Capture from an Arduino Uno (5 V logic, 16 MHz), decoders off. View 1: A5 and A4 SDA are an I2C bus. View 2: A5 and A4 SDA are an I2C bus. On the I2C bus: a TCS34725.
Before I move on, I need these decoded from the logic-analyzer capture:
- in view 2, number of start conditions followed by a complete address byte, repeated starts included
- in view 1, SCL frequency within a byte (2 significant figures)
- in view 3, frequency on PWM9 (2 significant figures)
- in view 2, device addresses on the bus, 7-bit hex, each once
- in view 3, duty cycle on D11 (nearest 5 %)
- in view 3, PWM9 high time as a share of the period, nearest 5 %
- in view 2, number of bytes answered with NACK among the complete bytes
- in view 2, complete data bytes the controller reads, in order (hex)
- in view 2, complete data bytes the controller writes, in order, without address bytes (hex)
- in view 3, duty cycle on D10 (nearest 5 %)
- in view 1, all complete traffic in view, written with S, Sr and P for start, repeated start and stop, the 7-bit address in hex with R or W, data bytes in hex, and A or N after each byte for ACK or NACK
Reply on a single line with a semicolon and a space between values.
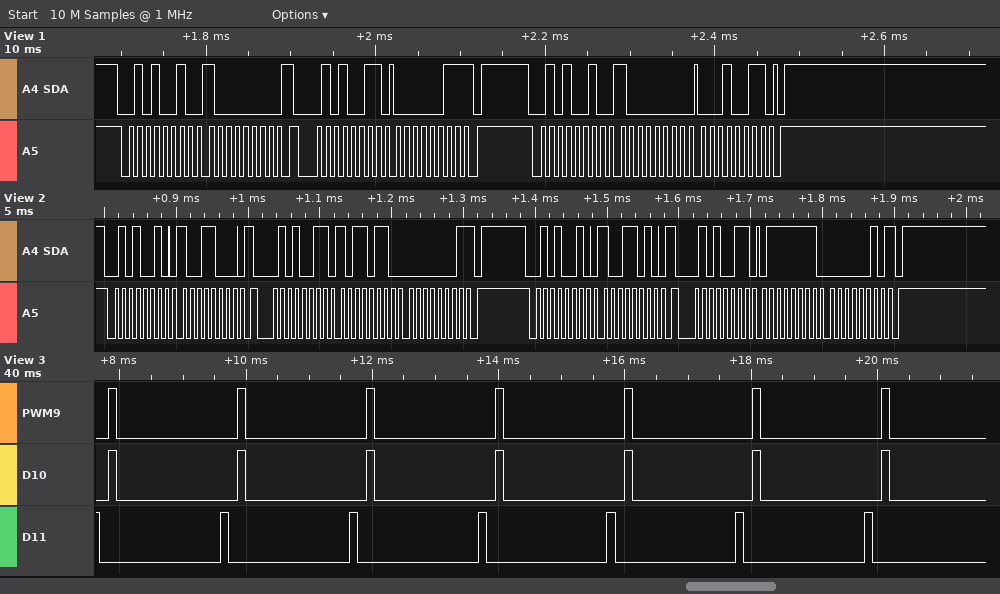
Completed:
4; 100 kHz; 490 Hz; 0x29; 5 %; 5 %; 2; B6 01 7F 02; 98 9A; 5 %; S 29W A 80 A Sr 29R A 03 N P S 29W A 80 A 13 A P
